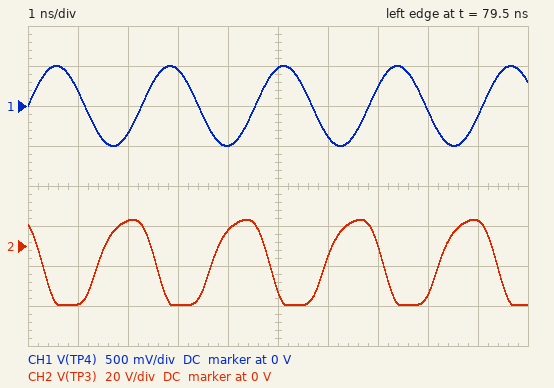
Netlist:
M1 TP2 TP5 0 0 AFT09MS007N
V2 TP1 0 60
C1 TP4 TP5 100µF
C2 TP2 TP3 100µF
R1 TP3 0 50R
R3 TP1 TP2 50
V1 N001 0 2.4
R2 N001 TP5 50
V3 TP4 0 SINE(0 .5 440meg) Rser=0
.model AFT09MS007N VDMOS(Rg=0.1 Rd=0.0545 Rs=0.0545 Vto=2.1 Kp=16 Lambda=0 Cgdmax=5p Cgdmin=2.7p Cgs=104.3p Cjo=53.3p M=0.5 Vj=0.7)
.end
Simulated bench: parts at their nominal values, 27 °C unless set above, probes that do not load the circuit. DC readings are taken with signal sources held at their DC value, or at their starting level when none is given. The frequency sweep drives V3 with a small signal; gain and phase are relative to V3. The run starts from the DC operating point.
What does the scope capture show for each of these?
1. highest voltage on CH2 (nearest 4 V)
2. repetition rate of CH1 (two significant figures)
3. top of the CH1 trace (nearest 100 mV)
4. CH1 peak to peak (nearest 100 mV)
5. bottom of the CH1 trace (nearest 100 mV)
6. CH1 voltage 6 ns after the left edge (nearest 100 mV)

12 V
440 MHz
500 mV
1.0 V
-500 mV
-400 mV
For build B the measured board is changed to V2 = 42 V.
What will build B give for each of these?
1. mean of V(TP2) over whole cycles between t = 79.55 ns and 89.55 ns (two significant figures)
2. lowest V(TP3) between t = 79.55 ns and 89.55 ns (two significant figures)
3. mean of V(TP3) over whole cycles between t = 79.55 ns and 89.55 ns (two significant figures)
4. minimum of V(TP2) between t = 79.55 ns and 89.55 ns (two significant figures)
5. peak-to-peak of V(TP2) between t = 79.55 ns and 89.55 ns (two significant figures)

10 V
-12 V
-1.9 V
210 mV
24 V
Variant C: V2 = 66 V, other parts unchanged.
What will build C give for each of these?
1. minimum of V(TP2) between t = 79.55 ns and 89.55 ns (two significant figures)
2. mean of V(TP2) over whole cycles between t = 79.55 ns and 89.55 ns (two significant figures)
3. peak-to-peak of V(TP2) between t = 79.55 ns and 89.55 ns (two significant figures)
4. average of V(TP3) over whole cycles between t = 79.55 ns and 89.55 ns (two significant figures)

460 mV
25 V
49 V
-11 V
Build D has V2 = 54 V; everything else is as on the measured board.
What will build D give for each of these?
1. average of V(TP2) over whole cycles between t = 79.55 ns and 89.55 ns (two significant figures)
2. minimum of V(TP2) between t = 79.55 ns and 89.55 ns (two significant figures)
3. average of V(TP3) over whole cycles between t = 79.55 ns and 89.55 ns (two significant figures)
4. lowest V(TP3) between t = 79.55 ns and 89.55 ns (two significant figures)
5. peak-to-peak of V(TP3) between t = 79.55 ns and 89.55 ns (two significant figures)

17 V
320 mV
-6.8 V
-24 V
37 V
